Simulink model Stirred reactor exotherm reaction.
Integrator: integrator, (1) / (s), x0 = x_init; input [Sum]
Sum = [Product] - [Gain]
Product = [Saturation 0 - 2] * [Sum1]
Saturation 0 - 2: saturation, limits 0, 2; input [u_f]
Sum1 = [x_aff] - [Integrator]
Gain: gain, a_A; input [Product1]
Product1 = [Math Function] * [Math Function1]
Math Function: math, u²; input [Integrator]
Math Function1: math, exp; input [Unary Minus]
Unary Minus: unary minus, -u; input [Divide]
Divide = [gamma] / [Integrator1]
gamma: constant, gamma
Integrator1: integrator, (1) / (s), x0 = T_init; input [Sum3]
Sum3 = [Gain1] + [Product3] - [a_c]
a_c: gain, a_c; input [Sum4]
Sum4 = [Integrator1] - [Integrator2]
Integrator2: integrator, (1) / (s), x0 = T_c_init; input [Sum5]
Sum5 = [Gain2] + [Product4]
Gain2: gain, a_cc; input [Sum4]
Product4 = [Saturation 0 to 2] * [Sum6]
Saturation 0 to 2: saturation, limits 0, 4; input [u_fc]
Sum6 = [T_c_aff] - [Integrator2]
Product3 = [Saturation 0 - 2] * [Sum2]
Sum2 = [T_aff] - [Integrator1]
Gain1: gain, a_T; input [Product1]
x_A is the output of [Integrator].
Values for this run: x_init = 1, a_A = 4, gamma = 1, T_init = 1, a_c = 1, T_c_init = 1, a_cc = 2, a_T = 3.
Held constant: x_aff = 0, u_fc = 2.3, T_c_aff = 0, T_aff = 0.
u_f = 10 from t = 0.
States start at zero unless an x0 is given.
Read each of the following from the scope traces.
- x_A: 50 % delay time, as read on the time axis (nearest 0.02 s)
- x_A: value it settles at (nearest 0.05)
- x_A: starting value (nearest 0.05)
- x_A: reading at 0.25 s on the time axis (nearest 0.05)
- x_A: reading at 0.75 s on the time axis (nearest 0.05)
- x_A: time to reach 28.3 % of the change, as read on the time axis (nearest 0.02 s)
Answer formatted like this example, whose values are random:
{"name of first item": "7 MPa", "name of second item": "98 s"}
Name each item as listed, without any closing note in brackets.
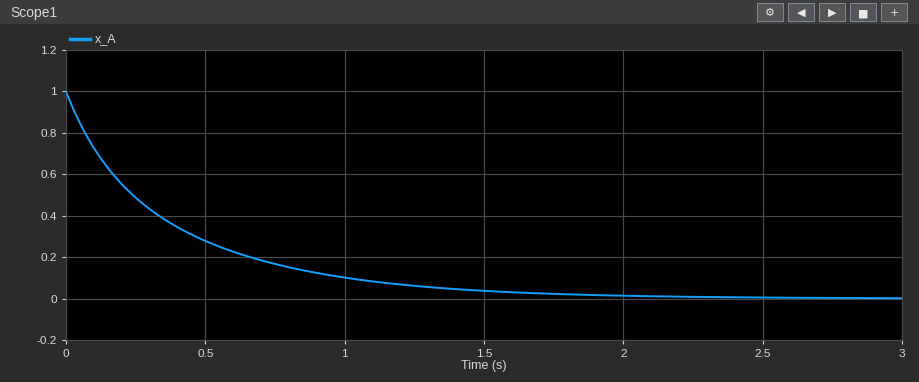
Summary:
{"x_A: 50 % delay time, as read on the time axis": "0.24 s", "x_A: value it settles at": "0.00", "x_A: starting value": "1.00", "x_A: reading at 0.25 s on the time axis": "0.50", "x_A: reading at 0.75 s on the time axis": "0.15", "x_A: time to reach 28.3 % of the change, as read on the time axis": "0.10 s"}
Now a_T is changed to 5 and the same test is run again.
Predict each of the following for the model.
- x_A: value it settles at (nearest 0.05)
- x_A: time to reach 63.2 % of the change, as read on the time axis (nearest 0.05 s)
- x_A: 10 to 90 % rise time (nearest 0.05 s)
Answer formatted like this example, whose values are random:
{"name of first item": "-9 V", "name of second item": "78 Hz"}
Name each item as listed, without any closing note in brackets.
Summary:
{"x_A: value it settles at": "0.00", "x_A: time to reach 63.2 % of the change, as read on the time axis": "0.35 s", "x_A: 10 to 90 % rise time": "0.95 s"}
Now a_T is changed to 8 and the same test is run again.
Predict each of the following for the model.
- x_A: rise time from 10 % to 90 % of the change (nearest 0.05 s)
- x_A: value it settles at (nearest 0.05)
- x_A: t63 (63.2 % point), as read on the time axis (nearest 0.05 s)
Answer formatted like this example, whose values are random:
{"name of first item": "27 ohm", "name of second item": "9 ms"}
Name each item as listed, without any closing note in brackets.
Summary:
{"x_A: rise time from 10 % to 90 % of the change": "0.95 s", "x_A: value it settles at": "0.00", "x_A: t63 (63.2 % point), as read on the time axis": "0.35 s"}
